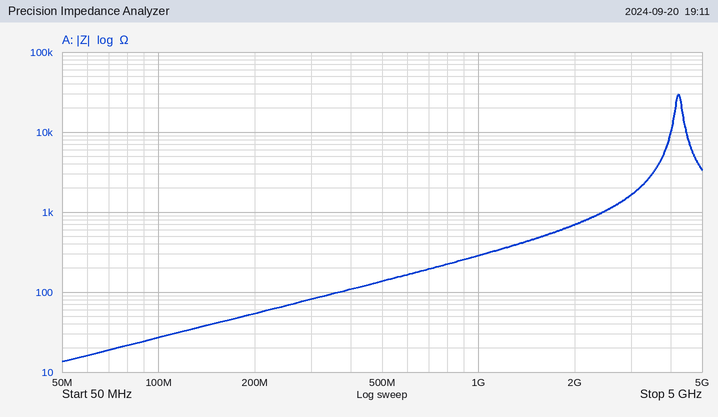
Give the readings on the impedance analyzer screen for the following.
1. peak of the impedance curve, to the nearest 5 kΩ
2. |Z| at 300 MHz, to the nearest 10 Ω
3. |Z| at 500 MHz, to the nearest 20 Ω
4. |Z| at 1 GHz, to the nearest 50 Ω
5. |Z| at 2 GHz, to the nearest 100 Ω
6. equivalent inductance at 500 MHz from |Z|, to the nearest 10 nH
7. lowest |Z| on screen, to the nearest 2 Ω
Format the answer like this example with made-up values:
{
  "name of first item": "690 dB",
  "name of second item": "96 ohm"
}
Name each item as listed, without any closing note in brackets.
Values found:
{
  "peak of the impedance curve, to the nearest 5 kΩ": "30 kΩ",
  "|Z| at 300 MHz, to the nearest 10 Ω": "80 Ω",
  "|Z| at 500 MHz, to the nearest 20 Ω": "140 Ω",
  "|Z| at 1 GHz, to the nearest 50 Ω": "300 Ω",
  "|Z| at 2 GHz, to the nearest 100 Ω": "700 Ω",
  "equivalent inductance at 500 MHz from |Z|, to the nearest 10 nH": "40 nH",
  "lowest |Z| on screen, to the nearest 2 Ω": "14 Ω"
}
